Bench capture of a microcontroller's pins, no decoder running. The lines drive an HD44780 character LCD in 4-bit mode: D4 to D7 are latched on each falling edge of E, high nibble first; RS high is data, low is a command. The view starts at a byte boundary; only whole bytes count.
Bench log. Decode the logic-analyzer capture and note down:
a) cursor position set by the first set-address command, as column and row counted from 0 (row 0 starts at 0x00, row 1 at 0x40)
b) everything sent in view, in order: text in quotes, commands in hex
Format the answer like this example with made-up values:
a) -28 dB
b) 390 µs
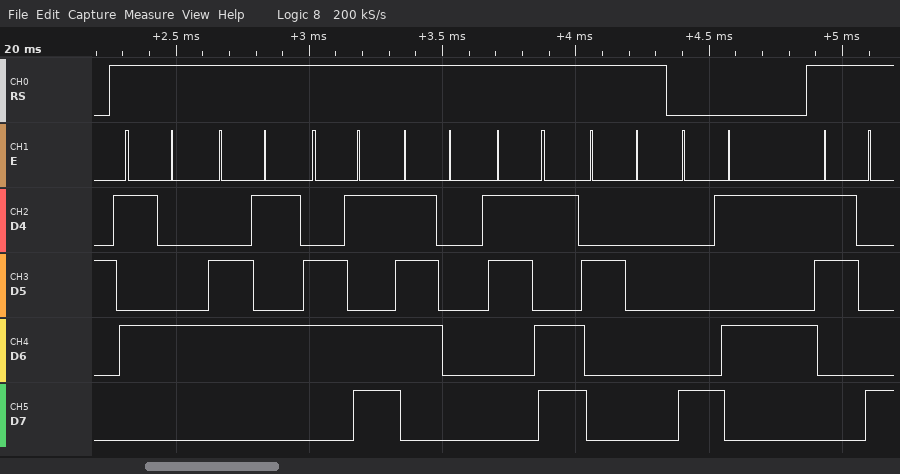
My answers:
a) column 5, row 0
b) "Temp= " 0x85 "8"
